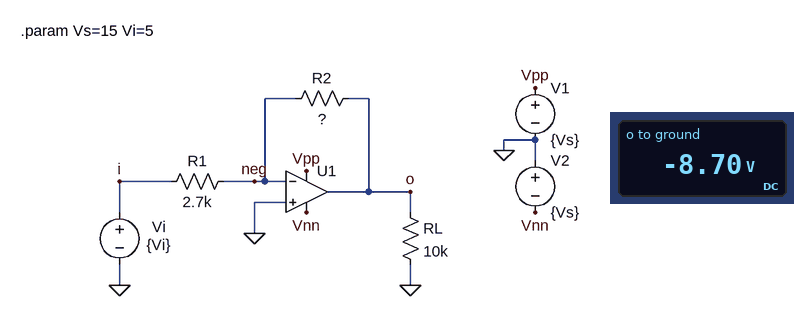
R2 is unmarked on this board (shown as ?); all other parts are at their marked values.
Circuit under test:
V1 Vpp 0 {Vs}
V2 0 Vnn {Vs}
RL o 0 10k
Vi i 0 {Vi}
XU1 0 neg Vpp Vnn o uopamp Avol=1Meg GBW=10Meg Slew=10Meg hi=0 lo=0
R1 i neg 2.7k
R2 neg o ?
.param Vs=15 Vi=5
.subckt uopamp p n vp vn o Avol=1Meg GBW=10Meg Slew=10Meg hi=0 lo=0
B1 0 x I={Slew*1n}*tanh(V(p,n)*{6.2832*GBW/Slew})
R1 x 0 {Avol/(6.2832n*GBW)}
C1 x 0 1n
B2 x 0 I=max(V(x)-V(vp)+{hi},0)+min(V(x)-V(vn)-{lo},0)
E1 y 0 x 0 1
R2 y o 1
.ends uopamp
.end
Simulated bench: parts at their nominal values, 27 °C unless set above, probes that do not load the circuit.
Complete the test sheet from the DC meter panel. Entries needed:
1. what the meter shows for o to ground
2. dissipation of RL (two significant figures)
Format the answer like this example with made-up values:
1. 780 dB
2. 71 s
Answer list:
1. -8.70 V
2. 7.6 mW
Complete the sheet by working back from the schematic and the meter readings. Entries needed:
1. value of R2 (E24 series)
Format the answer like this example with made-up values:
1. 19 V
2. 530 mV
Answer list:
1. 4.7 kΩ
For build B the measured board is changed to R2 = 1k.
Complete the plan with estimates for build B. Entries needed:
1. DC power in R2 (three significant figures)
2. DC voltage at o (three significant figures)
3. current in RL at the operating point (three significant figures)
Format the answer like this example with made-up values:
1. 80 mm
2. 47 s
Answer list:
1. 3.43 mW
2. -1.85 V
3. 185 µA
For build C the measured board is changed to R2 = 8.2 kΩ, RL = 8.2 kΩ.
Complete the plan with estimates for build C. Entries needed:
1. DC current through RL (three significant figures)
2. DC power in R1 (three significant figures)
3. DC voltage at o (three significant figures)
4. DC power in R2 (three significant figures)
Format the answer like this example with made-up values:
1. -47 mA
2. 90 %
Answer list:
1. 1.83 mA
2. 9.09 mW
3. -15.0 V
4. 27.6 mW
